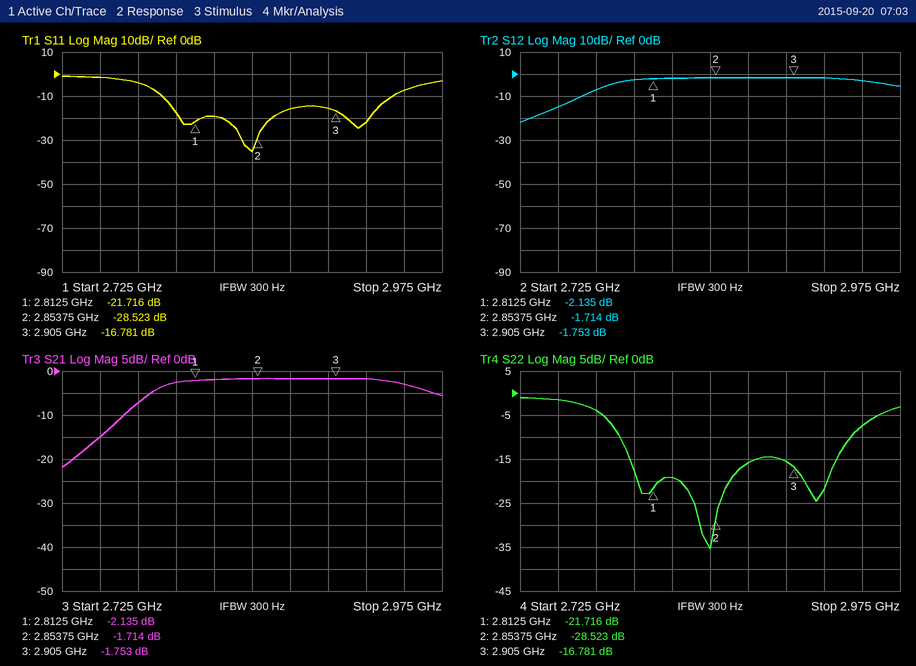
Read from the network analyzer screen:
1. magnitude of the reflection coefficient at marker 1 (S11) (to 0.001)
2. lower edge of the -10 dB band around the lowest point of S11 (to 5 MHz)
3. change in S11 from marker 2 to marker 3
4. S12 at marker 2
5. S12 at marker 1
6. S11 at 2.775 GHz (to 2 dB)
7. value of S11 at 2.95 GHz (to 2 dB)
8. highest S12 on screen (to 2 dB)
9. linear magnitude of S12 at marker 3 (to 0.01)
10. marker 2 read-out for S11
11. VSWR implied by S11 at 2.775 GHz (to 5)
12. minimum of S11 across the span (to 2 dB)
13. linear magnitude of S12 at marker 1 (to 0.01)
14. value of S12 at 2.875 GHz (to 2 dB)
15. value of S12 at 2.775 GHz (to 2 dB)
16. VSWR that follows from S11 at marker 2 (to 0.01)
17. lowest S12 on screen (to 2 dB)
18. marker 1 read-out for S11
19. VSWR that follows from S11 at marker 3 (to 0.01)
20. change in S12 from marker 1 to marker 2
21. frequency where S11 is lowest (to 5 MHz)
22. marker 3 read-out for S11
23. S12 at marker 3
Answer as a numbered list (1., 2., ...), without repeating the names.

1. 0.082
2. 2.790 GHz
3. 11.742 dB
4. -1.714 dB
5. -2.135 dB
6. -4 dB
7. -8 dB
8. -2 dB
9. 0.82
10. -28.523 dB
11. 5
12. -36 dB
13. 0.78
14. -2 dB
15. -8 dB
16. 1.08
17. -22 dB
18. -21.716 dB
19. 1.34
20. 0.421 dB
21. 2.850 GHz
22. -16.781 dB
23. -1.753 dB
